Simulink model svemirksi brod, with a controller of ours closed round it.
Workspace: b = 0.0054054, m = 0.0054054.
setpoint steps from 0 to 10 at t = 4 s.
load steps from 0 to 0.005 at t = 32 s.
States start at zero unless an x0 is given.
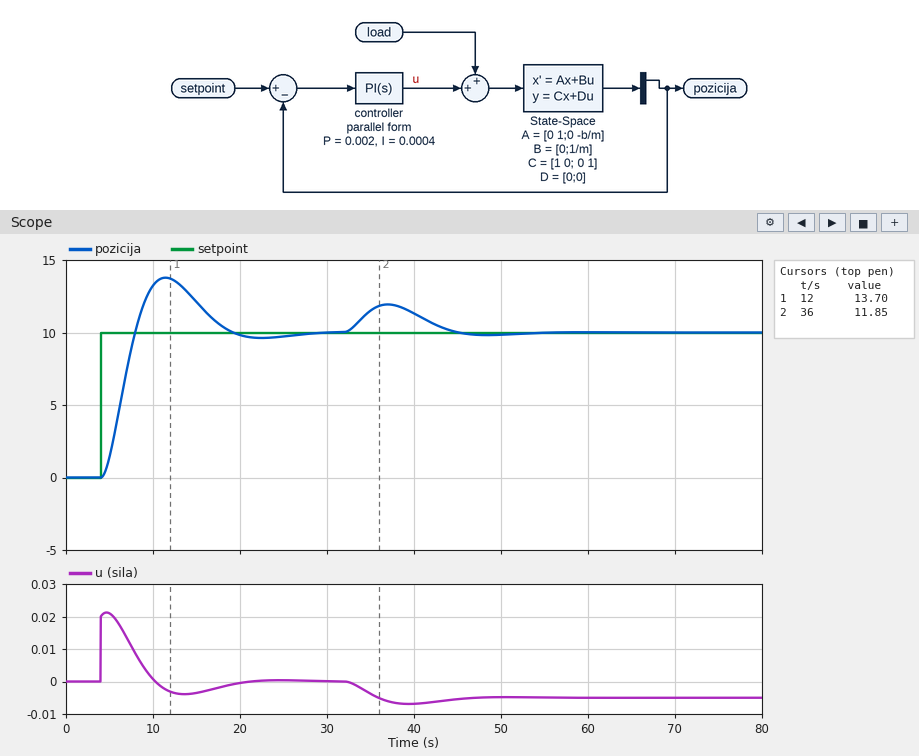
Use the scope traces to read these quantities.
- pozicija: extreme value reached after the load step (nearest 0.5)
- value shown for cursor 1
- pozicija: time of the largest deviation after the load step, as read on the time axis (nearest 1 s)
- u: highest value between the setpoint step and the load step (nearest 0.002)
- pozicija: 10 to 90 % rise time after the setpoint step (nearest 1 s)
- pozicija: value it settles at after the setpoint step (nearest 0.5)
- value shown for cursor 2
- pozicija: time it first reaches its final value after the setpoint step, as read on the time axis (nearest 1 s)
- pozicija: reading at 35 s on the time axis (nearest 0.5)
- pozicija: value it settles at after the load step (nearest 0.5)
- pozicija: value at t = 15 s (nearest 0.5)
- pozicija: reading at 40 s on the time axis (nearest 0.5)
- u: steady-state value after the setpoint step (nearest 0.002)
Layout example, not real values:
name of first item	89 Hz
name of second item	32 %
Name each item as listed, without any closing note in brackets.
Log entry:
pozicija: extreme value reached after the load step	12.0
value shown for cursor 1	13.70
pozicija: time of the largest deviation after the load step, as read on the time axis	37 s
u: highest value between the setpoint step and the load step	0.022
pozicija: 10 to 90 % rise time after the setpoint step	3 s
pozicija: value it settles at after the setpoint step	10.0
value shown for cursor 2	11.85
pozicija: time it first reaches its final value after the setpoint step, as read on the time axis	8 s
pozicija: reading at 35 s on the time axis	11.5
pozicija: value it settles at after the load step	10.0
pozicija: value at t = 15 s	12.0
pozicija: reading at 40 s on the time axis	11.5
u: steady-state value after the setpoint step	0.000
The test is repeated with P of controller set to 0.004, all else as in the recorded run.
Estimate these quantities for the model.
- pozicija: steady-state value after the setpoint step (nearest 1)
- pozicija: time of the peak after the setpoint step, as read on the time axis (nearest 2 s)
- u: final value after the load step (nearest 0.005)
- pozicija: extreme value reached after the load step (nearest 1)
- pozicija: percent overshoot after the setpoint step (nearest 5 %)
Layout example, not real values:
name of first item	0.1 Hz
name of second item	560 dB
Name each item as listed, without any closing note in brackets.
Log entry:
pozicija: steady-state value after the setpoint step	10
pozicija: time of the peak after the setpoint step, as read on the time axis	8 s
u: final value after the load step	-0.005
pozicija: extreme value reached after the load step	11
pozicija: percent overshoot after the setpoint step	25 %
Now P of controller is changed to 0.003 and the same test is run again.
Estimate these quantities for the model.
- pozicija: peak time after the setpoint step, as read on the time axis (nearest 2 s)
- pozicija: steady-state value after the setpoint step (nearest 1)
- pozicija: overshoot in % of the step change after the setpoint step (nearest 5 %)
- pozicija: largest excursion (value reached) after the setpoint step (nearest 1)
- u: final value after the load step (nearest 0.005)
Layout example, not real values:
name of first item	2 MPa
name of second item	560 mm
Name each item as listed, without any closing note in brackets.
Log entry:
pozicija: peak time after the setpoint step, as read on the time axis	10 s
pozicija: steady-state value after the setpoint step	10
pozicija: overshoot in % of the step change after the setpoint step	30 %
pozicija: largest excursion (value reached) after the setpoint step	13
u: final value after the load step	-0.005
